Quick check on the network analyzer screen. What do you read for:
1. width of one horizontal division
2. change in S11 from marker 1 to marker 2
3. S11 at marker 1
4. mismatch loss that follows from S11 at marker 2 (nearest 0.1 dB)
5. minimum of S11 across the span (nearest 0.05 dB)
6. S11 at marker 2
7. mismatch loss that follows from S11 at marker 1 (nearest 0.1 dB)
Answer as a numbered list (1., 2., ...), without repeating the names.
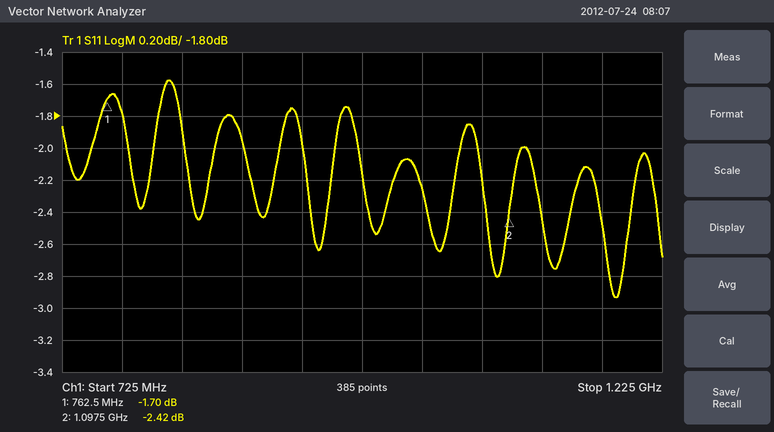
1. 50 MHz
2. -0.72 dB
3. -1.70 dB
4. 3.7 dB
5. -2.95 dB
6. -2.42 dB
7. 4.9 dB
